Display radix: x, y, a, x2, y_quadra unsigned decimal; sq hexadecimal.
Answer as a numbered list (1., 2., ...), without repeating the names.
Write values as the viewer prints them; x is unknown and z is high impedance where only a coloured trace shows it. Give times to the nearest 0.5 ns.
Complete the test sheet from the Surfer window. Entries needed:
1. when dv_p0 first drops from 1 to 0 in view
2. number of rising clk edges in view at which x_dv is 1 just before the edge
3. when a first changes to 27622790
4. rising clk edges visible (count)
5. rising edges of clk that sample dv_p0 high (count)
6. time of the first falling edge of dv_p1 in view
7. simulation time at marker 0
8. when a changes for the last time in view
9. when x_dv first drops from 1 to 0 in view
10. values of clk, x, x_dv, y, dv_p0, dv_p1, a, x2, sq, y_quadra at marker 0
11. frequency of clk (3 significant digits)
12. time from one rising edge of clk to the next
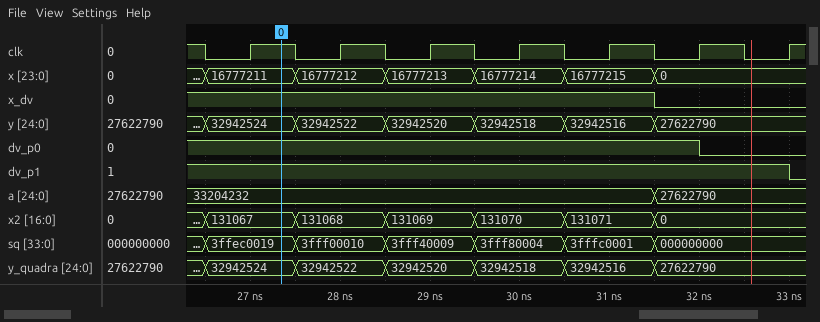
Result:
1. 32 ns
2. 5
3. 31.5 ns
4. 7
5. 6
6. 33 ns
7. 27.5 ns
8. 31.5 ns
9. 31.5 ns
10. clk=1, x=16777211, x_dv=1, y=32942524, dv_p0=1, dv_p1=1, a=33204232, x2=131067, sq=3ffec0019, y_quadra=32942524
11. 1.00 GHz
12. 1 ns
